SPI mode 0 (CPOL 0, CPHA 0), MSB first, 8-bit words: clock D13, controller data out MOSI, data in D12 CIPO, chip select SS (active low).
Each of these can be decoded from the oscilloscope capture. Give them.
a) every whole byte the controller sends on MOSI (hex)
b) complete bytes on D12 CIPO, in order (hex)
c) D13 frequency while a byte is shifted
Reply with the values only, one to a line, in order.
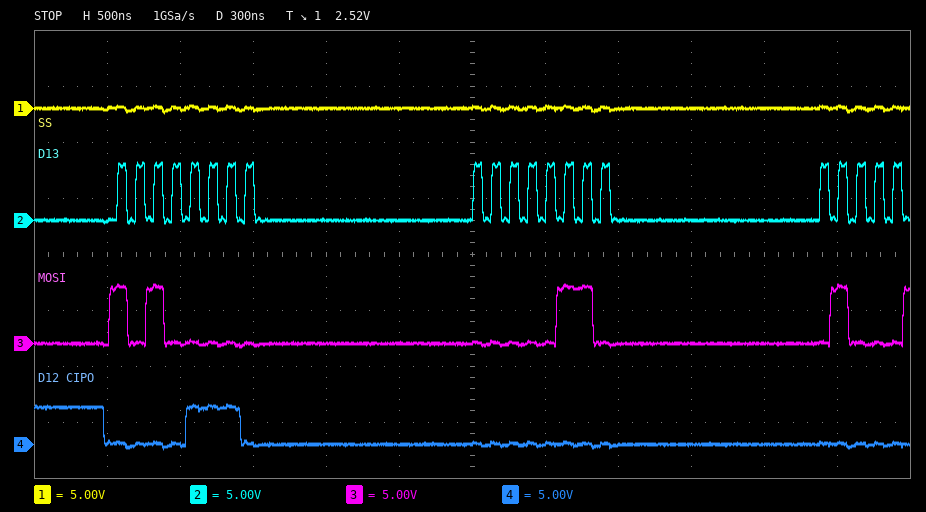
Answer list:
A0 06
0E 00
8 MHz
